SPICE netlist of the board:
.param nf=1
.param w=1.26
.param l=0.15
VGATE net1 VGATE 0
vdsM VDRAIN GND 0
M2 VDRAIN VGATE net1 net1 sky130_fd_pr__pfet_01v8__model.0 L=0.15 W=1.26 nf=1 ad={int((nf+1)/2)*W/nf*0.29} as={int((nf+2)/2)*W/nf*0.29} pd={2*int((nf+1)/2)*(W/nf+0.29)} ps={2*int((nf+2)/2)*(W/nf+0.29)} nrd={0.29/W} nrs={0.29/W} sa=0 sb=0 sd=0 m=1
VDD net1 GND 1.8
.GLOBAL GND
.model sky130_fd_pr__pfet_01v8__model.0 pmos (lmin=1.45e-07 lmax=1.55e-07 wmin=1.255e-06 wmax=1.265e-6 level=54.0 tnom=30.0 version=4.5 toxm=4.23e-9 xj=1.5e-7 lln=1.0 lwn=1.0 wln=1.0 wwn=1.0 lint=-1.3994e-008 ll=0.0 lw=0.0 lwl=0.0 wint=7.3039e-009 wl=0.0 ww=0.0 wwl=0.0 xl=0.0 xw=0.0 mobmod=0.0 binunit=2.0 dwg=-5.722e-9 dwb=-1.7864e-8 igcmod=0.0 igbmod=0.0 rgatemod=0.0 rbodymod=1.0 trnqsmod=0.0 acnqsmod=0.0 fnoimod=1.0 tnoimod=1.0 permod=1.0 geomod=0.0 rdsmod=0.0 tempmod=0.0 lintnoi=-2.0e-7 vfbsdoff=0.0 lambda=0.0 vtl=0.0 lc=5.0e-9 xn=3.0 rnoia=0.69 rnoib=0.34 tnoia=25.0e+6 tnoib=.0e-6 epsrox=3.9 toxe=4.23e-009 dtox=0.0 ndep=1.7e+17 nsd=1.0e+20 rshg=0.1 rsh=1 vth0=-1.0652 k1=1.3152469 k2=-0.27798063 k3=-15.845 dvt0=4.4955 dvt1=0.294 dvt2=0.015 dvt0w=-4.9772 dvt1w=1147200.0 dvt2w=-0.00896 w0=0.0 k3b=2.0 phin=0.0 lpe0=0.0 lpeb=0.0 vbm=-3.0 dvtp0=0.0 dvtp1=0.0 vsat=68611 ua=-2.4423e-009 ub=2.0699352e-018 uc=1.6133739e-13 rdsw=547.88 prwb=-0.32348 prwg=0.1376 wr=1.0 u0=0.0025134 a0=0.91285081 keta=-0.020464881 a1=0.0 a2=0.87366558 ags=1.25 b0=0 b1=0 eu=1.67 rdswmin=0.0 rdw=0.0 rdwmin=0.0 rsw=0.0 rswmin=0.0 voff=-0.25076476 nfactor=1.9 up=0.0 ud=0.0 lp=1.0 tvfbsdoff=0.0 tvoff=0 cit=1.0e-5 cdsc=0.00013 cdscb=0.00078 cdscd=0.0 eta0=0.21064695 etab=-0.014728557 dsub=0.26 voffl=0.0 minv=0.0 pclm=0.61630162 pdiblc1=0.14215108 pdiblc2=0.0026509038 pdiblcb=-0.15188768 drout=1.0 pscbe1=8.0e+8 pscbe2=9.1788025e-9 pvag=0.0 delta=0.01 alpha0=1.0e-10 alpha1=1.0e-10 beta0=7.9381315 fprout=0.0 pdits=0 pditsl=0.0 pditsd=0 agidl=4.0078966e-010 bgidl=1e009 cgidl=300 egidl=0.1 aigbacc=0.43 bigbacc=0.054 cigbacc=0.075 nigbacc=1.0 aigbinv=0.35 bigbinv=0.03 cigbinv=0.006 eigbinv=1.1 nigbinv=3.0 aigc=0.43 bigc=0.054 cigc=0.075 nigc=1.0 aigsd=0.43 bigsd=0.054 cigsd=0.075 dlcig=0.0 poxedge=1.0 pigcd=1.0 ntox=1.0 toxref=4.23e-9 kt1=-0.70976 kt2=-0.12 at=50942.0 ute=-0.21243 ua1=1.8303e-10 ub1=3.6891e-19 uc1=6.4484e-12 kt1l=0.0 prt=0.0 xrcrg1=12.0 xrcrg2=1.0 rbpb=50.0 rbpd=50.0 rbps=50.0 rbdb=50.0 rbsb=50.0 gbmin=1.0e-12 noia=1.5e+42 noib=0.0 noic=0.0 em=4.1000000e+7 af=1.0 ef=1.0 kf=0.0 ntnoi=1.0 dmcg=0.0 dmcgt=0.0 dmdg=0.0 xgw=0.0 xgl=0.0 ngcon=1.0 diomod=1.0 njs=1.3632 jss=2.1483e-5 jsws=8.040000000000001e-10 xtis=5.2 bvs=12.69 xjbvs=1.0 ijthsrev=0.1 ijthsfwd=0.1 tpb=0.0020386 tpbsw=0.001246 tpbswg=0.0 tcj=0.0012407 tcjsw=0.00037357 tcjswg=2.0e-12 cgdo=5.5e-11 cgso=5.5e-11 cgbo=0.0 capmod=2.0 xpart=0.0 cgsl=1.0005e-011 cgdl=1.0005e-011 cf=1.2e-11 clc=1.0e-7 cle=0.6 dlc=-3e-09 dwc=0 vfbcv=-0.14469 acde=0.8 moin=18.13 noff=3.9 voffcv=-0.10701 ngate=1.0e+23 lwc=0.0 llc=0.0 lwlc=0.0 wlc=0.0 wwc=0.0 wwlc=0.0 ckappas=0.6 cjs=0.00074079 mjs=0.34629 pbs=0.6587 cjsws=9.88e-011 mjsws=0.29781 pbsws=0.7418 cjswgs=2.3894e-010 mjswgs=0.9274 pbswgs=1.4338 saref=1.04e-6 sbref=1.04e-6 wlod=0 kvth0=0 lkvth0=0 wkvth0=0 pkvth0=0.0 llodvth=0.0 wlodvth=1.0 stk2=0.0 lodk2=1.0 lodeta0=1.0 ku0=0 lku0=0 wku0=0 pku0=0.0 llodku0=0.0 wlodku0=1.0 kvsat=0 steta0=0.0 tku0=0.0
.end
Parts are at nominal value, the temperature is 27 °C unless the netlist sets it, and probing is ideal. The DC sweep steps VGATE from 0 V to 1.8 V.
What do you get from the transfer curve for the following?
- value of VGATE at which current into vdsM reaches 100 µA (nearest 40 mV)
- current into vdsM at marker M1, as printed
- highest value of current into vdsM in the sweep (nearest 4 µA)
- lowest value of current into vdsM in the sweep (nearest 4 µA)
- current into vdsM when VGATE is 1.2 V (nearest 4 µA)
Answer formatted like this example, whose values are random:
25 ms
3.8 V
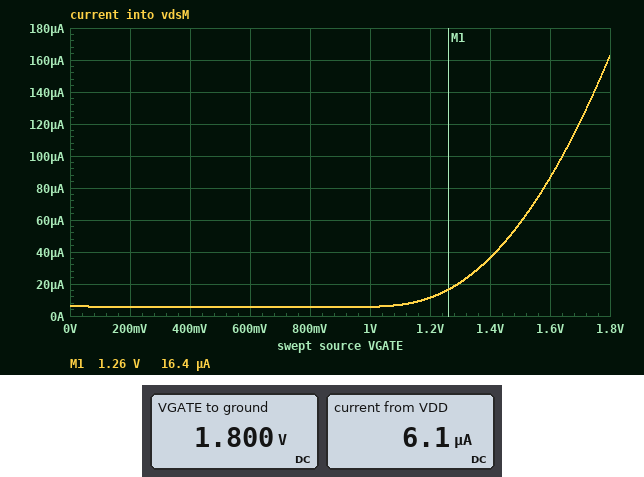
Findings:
1.64 V
16.4 µA
164 µA
4 µA
12 µA
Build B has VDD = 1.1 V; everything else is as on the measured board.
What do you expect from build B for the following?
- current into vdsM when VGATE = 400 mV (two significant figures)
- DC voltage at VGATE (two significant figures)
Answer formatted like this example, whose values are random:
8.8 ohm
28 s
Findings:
5.4 µA
1.1 V
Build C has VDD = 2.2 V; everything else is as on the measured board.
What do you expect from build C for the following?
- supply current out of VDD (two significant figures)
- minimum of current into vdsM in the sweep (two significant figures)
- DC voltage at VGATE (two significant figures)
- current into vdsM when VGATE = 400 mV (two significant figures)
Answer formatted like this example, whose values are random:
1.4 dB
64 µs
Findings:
12 µA
5.5 µA
2.2 V
6.7 µA
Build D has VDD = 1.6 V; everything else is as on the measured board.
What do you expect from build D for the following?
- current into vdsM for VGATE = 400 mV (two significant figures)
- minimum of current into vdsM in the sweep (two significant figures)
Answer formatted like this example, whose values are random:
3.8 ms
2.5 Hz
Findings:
5.4 µA
5.4 µA
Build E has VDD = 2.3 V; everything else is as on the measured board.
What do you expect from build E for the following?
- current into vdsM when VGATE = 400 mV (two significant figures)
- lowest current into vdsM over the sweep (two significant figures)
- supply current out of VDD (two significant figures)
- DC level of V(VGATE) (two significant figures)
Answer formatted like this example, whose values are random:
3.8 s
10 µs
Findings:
7.8 µA
5.6 µA
16 µA
2.3 V
